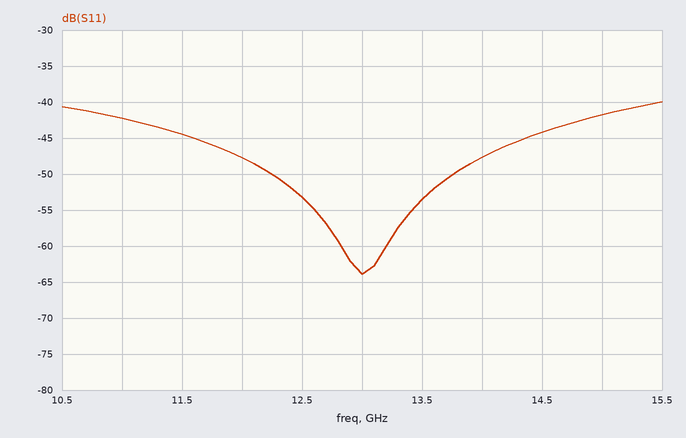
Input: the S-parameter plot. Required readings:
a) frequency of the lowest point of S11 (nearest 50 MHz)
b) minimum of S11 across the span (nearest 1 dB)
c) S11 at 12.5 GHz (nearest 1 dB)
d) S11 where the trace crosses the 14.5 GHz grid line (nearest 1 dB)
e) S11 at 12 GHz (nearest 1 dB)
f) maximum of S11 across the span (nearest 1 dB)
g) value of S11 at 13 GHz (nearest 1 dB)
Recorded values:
13.00 GHz
-64 dB
-53 dB
-44 dB
-48 dB
-40 dB
-64 dB
